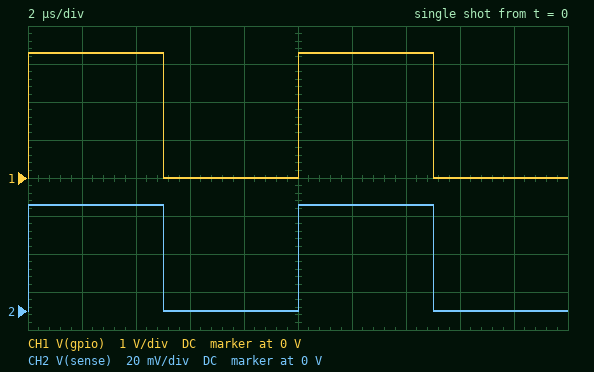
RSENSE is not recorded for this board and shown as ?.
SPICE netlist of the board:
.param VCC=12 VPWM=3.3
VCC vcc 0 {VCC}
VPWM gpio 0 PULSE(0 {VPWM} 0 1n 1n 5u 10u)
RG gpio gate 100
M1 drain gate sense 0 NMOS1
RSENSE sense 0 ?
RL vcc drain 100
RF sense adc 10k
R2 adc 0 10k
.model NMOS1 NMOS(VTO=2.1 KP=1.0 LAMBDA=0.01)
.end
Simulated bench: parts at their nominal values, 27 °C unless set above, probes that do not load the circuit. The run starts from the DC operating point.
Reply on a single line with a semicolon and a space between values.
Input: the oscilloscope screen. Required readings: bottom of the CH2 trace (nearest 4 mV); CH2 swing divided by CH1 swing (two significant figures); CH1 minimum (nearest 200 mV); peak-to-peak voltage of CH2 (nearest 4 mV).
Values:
0 V; 0.017; 0 V; 56 mV
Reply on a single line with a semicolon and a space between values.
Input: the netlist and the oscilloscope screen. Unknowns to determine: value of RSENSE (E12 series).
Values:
0.47 Ω
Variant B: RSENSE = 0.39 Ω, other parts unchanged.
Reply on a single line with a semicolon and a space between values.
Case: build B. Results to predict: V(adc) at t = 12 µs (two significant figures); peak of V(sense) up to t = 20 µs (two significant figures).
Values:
23 mV; 46 mV
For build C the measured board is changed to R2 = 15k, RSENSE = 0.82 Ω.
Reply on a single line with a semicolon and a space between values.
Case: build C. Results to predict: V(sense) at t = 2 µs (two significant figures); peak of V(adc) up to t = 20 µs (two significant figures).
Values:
97 mV; 58 mV
